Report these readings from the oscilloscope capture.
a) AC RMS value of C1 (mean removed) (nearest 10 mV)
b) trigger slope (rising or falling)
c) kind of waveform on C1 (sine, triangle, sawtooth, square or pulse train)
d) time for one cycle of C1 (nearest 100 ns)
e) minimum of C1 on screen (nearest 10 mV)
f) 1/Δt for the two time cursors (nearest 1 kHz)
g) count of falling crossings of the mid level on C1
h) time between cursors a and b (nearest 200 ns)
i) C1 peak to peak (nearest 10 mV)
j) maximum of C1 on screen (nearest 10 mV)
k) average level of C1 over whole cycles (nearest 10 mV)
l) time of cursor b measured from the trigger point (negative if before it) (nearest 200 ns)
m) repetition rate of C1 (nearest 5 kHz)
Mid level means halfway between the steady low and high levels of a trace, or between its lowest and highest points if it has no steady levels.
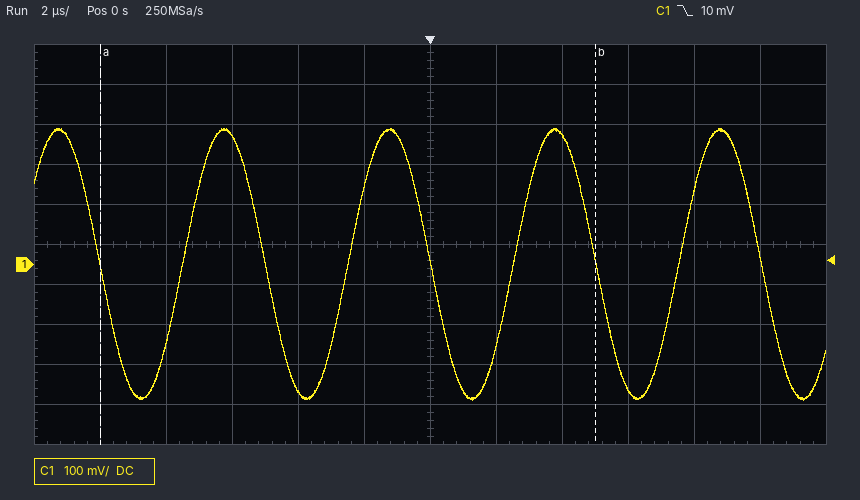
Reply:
240 mV
falling
sine
5.0 µs
-340 mV
67 kHz
5
15.0 µs
680 mV
340 mV
0 mV
+5.0 µs
200 kHz
